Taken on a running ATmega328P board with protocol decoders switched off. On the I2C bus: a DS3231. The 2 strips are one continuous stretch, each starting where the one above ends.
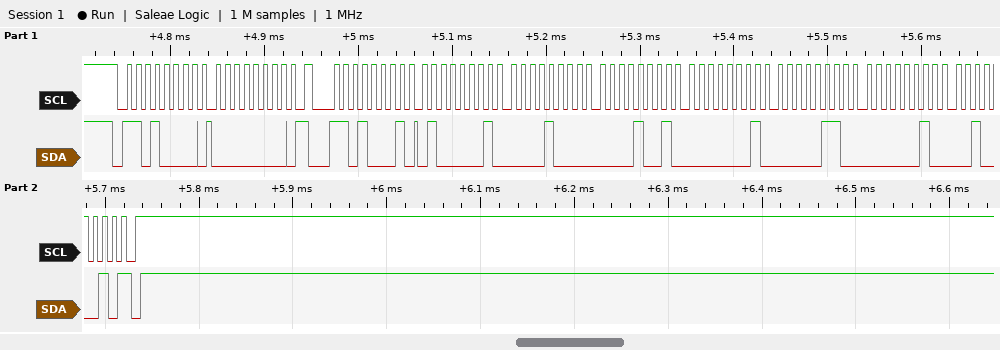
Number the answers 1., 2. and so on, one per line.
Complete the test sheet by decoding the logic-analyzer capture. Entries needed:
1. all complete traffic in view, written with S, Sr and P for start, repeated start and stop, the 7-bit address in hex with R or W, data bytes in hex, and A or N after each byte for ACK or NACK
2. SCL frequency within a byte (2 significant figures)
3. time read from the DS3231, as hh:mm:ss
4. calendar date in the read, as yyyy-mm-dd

1. S 68W A 00 A Sr 68R A 41 A 08 A 09 A 01 A 06 A 02 A 22 N P
2. 100 kHz
3. 09:08:41
4. 2022-02-06
